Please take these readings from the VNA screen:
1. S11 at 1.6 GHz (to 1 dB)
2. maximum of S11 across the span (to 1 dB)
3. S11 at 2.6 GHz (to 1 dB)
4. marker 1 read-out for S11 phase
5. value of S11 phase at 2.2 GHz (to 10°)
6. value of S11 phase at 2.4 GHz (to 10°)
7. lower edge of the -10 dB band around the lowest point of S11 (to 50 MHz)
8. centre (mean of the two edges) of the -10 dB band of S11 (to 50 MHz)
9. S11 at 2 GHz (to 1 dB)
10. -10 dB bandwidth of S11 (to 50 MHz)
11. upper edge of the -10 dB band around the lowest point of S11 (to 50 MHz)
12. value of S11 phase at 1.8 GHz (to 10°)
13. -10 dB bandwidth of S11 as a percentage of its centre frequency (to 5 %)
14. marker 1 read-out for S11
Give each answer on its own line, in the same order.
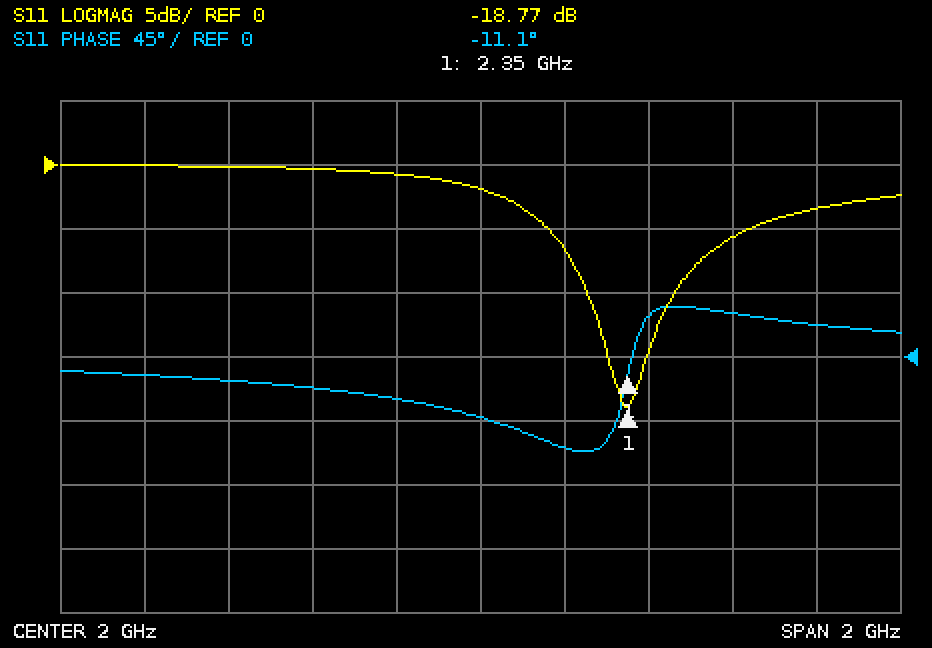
0 dB
0 dB
-6 dB
-11.1°
-60°
30°
2.25 GHz
2.35 GHz
-2 dB
200 MHz
2.45 GHz
-30°
10 %
-18.77 dB
